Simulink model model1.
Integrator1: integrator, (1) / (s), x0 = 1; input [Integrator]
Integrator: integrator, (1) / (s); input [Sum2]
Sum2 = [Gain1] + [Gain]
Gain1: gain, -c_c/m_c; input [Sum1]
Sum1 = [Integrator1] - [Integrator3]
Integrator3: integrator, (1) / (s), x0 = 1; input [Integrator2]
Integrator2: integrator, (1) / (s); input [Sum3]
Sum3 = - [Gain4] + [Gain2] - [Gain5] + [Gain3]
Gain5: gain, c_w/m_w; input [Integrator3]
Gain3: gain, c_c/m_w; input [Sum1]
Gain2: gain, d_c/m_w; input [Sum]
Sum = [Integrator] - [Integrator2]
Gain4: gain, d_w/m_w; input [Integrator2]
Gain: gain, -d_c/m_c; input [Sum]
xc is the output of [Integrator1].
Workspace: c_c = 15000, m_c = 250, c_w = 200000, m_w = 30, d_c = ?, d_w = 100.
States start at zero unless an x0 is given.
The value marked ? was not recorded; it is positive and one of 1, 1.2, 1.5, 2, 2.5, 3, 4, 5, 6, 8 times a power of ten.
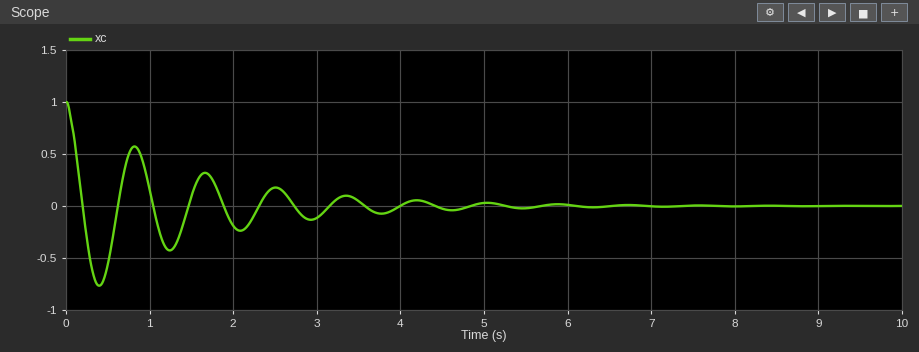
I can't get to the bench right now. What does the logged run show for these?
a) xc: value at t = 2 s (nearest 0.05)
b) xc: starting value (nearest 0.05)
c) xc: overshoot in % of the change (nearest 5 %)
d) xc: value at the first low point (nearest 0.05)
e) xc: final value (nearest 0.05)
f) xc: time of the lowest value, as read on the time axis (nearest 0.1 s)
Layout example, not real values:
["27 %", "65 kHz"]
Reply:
["-0.20", "1.00", "75 %", "-0.75", "0.00", "0.4 s"]
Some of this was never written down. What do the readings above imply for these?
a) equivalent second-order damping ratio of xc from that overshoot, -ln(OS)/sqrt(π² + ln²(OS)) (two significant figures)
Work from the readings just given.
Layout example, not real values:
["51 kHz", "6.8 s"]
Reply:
["0.091"]
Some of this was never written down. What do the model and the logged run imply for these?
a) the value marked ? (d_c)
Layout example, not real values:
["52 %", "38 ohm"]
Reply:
["400"]
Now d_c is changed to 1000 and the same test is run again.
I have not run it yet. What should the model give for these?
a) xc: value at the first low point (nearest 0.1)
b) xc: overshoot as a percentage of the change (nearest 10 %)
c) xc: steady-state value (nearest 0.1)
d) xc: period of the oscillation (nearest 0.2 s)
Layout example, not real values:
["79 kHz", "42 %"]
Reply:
["-0.5", "50 %", "0.0", "0.8 s"]
